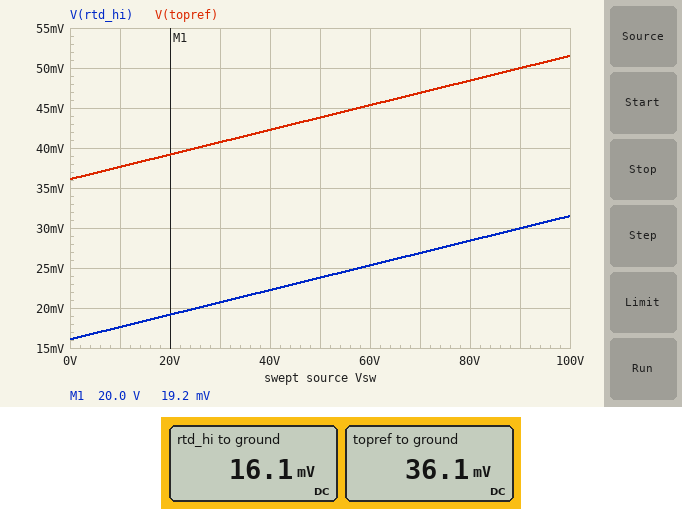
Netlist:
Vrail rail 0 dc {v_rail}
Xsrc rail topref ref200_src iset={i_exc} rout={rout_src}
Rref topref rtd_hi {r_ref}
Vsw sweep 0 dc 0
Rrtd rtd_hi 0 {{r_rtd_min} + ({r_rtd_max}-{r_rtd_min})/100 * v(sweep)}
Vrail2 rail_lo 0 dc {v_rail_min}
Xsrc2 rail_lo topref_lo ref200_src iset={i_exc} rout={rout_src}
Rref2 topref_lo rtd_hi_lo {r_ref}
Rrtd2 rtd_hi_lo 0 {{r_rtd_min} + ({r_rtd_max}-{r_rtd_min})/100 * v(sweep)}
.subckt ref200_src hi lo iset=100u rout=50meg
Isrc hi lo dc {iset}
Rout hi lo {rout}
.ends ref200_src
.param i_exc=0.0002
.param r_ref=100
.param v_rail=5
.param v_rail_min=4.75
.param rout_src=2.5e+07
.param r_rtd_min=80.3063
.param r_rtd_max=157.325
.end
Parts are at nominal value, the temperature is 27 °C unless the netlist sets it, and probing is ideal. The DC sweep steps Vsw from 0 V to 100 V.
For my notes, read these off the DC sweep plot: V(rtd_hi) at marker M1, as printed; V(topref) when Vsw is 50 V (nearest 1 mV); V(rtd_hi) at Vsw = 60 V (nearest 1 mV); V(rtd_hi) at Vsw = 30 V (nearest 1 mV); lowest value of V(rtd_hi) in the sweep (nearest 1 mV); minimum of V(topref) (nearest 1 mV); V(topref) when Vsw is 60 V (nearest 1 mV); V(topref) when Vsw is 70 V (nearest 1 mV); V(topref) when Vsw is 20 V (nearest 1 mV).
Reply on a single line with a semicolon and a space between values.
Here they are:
19.2 mV; 44 mV; 25 mV; 21 mV; 16 mV; 36 mV; 45 mV; 47 mV; 39 mV
